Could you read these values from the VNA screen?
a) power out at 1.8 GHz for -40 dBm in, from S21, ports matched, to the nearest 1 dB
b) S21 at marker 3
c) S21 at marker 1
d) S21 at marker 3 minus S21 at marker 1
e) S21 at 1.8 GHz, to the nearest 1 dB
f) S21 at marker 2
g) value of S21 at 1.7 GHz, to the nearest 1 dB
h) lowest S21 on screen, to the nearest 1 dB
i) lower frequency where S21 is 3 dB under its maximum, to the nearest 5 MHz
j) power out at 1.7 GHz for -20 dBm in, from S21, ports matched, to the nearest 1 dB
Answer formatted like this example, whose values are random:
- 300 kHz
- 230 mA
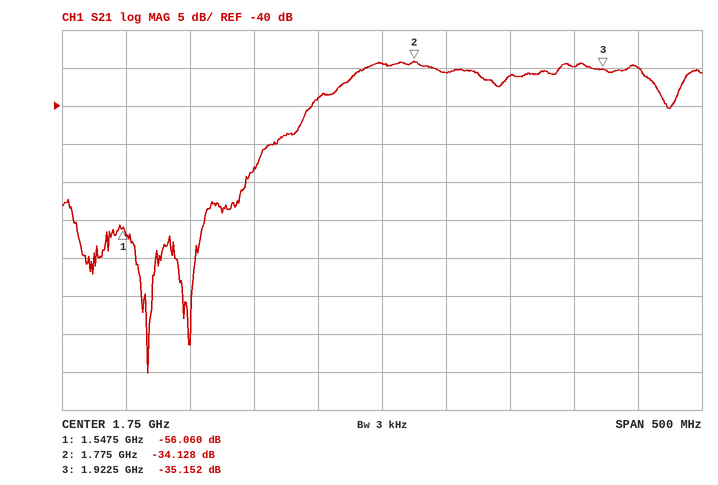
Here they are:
- -76 dBm
- -35.152 dB
- -56.060 dB
- 20.908 dB
- -36 dB
- -34.128 dB
- -39 dB
- -75 dB
- 1.720 GHz
- -59 dBm
